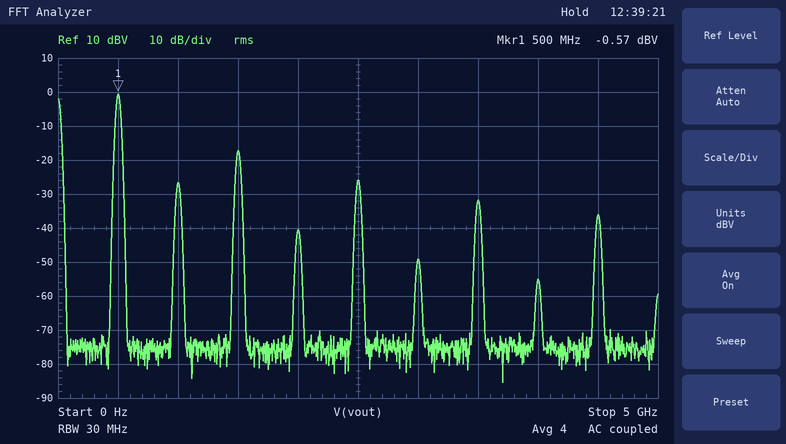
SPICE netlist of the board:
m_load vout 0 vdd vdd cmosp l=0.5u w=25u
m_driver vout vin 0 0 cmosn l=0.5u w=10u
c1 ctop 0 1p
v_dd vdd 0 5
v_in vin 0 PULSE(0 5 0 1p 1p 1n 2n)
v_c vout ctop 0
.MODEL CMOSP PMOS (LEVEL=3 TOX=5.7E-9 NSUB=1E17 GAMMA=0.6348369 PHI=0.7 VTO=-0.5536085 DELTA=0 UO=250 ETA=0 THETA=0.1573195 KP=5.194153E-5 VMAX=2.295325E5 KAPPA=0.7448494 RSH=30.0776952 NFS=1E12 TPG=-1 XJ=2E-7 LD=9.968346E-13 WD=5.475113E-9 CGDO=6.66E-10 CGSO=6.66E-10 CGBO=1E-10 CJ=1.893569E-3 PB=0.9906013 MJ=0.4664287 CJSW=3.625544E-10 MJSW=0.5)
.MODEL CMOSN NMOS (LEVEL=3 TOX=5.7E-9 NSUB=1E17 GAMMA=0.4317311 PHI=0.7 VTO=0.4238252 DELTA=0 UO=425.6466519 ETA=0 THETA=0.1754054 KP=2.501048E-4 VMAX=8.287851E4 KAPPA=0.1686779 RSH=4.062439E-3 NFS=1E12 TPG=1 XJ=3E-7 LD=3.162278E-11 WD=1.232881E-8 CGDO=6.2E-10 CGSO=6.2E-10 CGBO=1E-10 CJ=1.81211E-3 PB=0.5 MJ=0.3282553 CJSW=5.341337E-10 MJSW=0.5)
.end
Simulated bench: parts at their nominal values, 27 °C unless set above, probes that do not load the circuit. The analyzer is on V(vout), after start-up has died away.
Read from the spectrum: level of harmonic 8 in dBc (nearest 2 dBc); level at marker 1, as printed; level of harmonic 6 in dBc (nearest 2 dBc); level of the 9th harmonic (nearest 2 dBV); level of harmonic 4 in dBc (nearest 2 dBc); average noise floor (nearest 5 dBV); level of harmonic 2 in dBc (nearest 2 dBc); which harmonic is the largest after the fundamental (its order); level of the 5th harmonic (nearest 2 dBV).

-54 dBc
-0.57 dBV
-48 dBc
-36 dBV
-40 dBc
-75 dBV
-26 dBc
3
-26 dBV
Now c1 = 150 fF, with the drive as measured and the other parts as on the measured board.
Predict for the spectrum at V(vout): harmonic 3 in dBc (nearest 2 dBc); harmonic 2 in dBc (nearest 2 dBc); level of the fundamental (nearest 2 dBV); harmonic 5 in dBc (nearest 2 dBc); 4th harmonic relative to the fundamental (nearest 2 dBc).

-12 dBc
-24 dBc
4 dBV
-18 dBc
-28 dBc
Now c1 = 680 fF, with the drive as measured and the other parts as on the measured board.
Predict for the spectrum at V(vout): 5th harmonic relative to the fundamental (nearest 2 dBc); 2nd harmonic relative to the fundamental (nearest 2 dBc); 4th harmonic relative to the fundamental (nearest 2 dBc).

-24 dBc
-24 dBc
-36 dBc
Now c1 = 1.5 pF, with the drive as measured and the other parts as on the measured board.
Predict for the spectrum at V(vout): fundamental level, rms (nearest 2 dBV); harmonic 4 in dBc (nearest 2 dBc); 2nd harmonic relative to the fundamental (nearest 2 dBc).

-2 dBV
-44 dBc
-30 dBc
